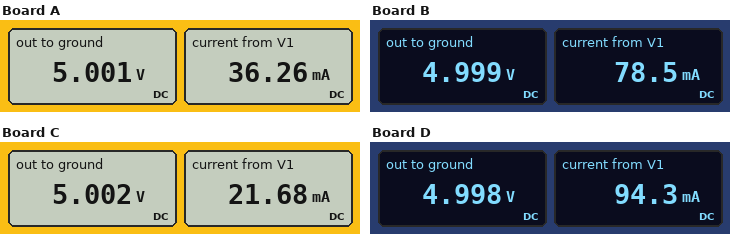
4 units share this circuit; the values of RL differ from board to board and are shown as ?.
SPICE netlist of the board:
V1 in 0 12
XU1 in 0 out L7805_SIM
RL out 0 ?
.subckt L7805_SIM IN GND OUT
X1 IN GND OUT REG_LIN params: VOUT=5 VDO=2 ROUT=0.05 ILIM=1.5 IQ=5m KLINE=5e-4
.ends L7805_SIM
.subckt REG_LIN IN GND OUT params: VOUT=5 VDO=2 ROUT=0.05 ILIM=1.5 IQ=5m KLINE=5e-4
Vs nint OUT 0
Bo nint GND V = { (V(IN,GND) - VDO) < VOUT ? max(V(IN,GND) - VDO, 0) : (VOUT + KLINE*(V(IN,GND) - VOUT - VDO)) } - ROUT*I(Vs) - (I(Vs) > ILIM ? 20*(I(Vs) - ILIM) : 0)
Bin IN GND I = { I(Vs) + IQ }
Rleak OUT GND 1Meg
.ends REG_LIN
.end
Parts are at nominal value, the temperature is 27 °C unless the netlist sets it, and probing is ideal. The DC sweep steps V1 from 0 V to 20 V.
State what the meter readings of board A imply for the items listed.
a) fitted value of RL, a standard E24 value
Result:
160 Ω
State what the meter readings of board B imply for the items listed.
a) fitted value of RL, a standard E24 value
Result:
68 Ω
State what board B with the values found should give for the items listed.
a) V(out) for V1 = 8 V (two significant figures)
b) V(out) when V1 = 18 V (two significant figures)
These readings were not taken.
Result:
5.0 V
5.0 V
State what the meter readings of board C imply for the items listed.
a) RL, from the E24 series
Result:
300 Ω
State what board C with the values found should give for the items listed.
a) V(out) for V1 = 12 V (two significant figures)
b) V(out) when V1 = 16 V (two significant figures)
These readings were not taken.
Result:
5.0 V
5.0 V
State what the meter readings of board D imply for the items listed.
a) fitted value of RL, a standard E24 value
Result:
56 Ω
